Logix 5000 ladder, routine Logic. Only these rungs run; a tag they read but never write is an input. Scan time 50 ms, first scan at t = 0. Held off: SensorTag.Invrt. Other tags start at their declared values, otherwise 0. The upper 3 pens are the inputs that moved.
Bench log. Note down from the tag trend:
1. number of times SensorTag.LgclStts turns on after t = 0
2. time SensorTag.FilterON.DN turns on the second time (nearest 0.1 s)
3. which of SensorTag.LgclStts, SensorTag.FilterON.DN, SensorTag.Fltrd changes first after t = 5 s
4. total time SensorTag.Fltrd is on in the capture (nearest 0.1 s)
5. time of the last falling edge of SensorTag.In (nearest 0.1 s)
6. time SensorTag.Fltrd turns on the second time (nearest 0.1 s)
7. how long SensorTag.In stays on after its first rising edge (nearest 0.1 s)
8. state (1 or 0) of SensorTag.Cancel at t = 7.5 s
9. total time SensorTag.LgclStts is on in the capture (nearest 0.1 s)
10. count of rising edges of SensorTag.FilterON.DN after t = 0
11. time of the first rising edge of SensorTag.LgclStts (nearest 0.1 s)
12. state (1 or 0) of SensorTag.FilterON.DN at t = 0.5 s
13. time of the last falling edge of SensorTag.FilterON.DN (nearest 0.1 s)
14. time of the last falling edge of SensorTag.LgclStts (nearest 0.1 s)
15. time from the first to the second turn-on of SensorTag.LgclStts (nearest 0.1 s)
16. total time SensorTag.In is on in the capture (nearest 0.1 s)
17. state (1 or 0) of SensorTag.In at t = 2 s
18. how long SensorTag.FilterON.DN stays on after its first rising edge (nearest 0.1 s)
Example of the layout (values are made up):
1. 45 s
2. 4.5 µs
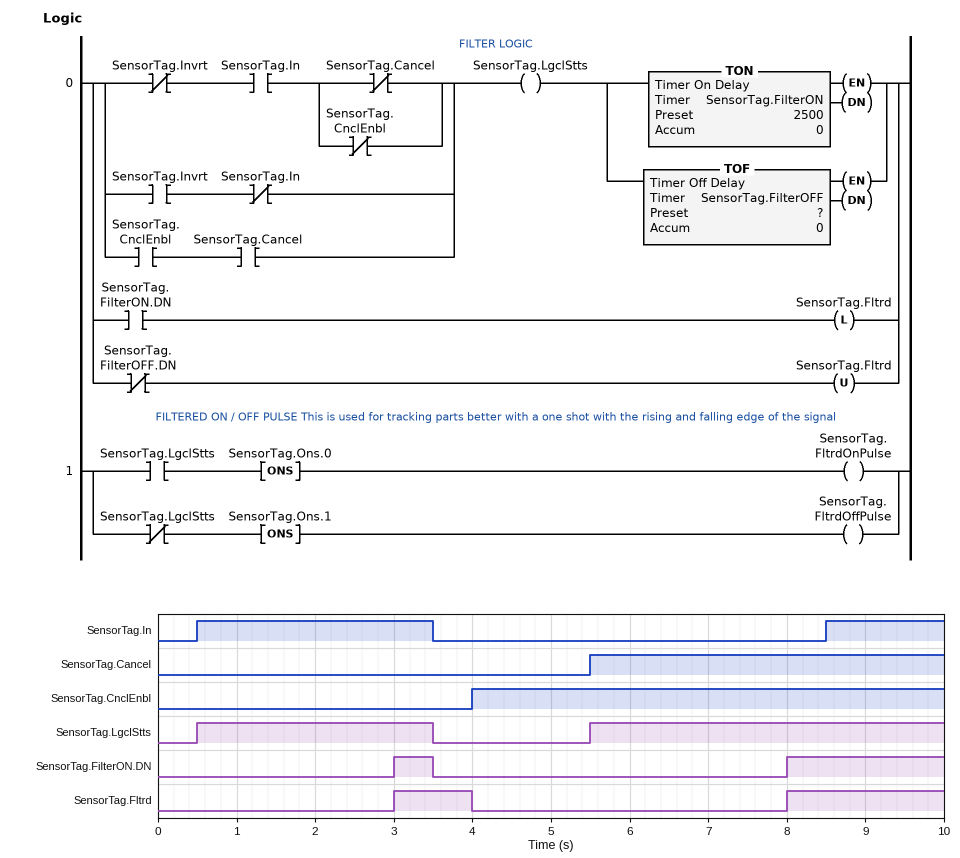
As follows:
1. 2
2. 8.0 s
3. SensorTag.LgclStts
4. 3.0 s
5. 3.5 s
6. 8.0 s
7. 3.0 s
8. 1
9. 7.5 s
10. 2
11. 0.5 s
12. 0
13. 3.5 s
14. 3.5 s
15. 5.0 s
16. 4.5 s
17. 1
18. 0.5 s
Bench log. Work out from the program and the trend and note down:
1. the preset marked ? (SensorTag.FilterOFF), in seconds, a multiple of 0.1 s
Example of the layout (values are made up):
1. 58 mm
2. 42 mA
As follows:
1. 0.5 s
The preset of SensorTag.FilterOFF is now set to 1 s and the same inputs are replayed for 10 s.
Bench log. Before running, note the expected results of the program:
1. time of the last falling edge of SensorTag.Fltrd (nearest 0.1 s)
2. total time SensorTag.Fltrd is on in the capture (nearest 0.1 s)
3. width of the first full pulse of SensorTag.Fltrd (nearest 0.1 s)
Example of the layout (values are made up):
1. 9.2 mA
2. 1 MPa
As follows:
1. 4.5 s
2. 3.5 s
3. 1.5 s
